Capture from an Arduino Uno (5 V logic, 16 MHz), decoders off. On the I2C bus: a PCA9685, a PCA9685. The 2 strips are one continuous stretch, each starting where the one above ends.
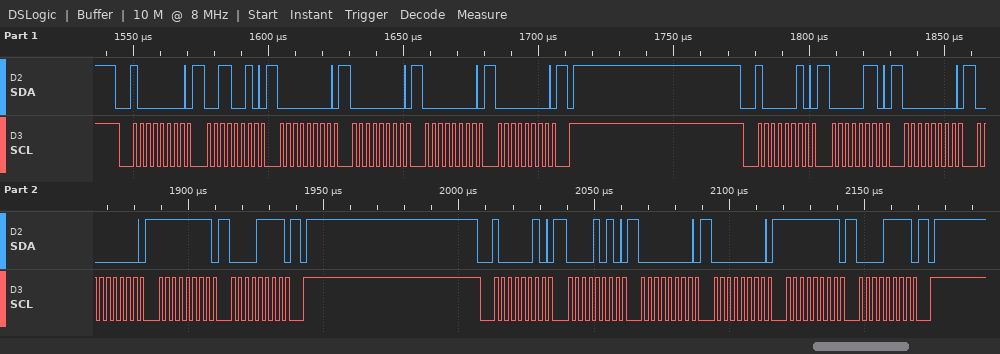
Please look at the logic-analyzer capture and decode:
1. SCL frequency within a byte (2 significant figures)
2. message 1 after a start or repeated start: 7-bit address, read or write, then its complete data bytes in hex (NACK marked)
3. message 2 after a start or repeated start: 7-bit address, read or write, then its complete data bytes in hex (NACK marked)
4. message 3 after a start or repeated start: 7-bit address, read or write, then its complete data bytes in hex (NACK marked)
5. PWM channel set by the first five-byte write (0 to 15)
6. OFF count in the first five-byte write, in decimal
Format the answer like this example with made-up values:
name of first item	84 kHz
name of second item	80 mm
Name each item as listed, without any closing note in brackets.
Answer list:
SCL frequency within a byte	400 kHz
message 1 after a start or repeated start: 7-bit address, read or write, then its complete data bytes in hex	0x40 write: 32 00 00 00 00
message 2 after a start or repeated start: 7-bit address, read or write, then its complete data bytes in hex	0x41 write: 06 00 00 FF 0F
message 3 after a start or repeated start: 7-bit address, read or write, then its complete data bytes in hex	0x41 write: 0A 00 00 FF 0F
PWM channel set by the first five-byte write	11
OFF count in the first five-byte write, in decimal	0
